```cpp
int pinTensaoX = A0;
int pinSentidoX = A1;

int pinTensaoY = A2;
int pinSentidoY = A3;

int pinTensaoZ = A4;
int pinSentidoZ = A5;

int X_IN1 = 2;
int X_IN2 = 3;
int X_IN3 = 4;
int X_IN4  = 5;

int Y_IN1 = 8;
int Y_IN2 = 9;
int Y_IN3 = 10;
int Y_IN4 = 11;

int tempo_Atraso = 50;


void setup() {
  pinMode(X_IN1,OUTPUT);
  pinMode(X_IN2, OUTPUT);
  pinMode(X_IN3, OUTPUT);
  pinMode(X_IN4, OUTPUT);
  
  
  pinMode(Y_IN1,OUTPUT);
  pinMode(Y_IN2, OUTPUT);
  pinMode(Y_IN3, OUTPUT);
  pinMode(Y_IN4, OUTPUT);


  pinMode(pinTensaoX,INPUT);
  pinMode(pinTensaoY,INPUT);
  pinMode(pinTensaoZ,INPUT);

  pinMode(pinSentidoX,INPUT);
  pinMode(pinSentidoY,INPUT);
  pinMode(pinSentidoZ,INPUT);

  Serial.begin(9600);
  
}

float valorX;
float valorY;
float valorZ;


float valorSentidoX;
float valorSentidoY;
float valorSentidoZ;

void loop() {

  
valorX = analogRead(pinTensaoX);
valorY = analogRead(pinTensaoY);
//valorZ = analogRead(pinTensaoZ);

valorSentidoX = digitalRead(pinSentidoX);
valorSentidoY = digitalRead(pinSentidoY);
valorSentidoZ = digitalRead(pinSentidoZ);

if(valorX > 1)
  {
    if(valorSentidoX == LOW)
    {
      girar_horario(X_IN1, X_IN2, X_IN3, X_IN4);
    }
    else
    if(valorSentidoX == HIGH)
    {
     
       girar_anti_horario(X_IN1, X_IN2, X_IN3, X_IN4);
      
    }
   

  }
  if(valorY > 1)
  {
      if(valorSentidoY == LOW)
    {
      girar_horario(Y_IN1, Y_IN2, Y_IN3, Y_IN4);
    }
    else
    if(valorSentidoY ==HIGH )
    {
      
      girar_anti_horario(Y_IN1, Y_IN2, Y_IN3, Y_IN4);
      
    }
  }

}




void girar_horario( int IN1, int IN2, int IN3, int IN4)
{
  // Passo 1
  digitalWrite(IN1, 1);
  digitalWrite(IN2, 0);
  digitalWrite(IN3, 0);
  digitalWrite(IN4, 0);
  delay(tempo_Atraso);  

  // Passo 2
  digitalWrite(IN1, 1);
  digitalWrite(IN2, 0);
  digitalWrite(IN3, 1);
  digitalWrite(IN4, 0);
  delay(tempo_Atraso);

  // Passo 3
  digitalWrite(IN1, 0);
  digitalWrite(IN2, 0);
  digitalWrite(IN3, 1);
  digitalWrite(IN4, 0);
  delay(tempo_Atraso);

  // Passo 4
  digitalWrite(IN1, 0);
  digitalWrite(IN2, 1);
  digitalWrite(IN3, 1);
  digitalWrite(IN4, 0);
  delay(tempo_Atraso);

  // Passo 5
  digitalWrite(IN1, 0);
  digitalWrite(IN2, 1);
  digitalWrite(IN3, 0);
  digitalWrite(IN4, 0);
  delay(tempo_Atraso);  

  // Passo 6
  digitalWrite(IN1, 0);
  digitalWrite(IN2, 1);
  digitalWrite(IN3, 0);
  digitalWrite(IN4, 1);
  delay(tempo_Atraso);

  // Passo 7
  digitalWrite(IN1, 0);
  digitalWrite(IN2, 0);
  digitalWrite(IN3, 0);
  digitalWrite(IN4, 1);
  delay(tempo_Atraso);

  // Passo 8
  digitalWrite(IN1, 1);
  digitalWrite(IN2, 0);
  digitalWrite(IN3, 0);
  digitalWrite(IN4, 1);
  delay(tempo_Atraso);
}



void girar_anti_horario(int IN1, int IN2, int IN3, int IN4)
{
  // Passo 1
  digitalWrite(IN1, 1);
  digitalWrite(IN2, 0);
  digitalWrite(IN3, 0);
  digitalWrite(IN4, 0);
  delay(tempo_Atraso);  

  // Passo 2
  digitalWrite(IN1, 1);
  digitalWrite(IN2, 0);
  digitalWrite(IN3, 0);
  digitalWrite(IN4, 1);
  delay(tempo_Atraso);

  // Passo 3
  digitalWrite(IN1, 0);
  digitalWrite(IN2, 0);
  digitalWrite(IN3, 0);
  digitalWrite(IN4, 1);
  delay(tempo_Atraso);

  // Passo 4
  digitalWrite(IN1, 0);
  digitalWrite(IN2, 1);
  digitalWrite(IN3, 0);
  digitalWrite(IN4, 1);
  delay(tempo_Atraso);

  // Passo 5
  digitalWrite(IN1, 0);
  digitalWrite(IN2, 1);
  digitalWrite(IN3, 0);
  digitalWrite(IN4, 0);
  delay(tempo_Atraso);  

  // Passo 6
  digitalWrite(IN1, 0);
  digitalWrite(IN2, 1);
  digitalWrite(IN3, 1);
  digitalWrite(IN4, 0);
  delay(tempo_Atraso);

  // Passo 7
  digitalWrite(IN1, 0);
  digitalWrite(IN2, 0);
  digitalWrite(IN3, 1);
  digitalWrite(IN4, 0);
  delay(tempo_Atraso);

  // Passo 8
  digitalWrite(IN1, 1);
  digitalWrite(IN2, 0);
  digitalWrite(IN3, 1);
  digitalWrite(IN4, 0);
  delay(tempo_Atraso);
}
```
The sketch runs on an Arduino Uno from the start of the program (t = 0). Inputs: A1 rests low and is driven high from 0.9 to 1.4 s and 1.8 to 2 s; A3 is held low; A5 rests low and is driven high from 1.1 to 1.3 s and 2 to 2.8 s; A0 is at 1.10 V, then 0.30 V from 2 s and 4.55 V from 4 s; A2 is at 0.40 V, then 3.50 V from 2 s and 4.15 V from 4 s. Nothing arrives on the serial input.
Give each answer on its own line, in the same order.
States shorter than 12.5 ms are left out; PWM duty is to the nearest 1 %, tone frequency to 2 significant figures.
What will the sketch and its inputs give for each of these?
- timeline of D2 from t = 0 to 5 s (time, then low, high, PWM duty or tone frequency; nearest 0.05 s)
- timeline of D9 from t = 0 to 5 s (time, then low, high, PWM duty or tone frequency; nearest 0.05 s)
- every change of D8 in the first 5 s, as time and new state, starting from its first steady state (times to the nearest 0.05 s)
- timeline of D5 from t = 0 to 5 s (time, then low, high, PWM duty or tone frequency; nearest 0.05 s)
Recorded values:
0 s high; 0.1 s low; 0.35 s high; 0.9 s low; 1.15 s high; 1.7 s low; 1.95 s high; 2.5 s low; 2.75 s high; 3.3 s low; 3.55 s high; 4.1 s low; 4.35 s high; 4.9 s low
0 s low; 0.55 s high; 0.7 s low; 1.35 s high; 1.5 s low; 2.15 s high; 2.3 s low; 2.95 s high; 3.1 s low; 3.75 s high; 3.9 s low; 4.55 s high; 4.7 s low
0 s low; 0.4 s high; 0.5 s low; 0.75 s high; 1.3 s low; 1.55 s high; 2.1 s low; 2.35 s high; 2.9 s low; 3.15 s high; 3.7 s low; 3.95 s high; 4.5 s low; 4.75 s high
0 s low; 0.25 s high; 0.8 s low; 1.05 s high; 1.6 s low; 1.85 s high; 2.4 s low; 2.65 s high; 3.2 s low; 3.45 s high; 4 s low; 4.25 s high; 4.8 s low
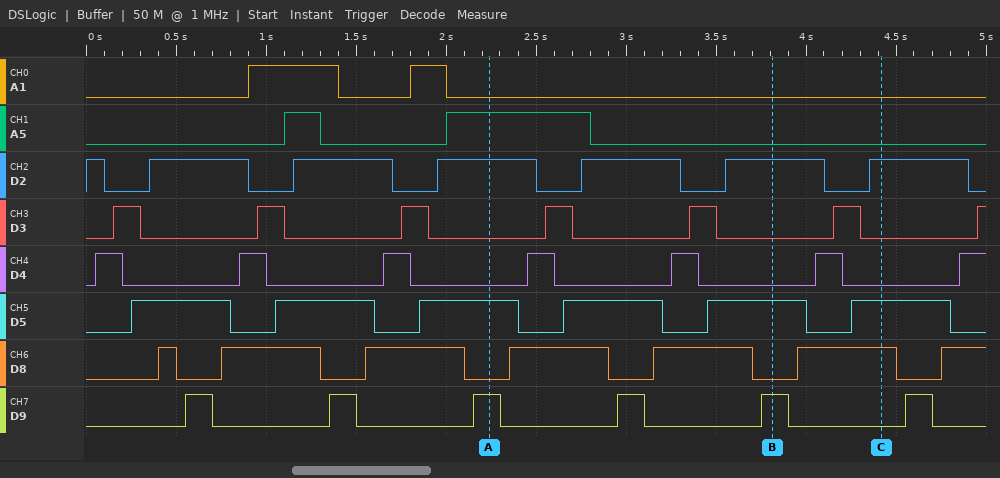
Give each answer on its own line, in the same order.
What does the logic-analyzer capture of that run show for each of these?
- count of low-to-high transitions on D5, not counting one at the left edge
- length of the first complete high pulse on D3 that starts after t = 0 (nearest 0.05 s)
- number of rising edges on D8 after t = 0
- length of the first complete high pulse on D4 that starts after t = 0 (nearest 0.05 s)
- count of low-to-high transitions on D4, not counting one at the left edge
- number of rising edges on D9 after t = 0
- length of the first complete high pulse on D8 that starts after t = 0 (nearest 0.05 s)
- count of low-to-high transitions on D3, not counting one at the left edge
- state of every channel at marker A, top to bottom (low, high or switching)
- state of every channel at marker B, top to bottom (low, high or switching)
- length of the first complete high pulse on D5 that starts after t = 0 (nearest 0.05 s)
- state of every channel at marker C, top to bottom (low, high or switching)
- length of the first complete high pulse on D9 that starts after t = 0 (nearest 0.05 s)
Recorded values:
6
0.15 s
7
0.15 s
7
6
0.10 s
7
A1 low, A5 high, D2 high, D3 low, D4 low, D5 high, D8 low, D9 high
A1 low, A5 low, D2 high, D3 low, D4 low, D5 high, D8 low, D9 high
0.55 s
A1 low, A5 low, D2 high, D3 low, D4 low, D5 high, D8 high, D9 low
0.15 s
